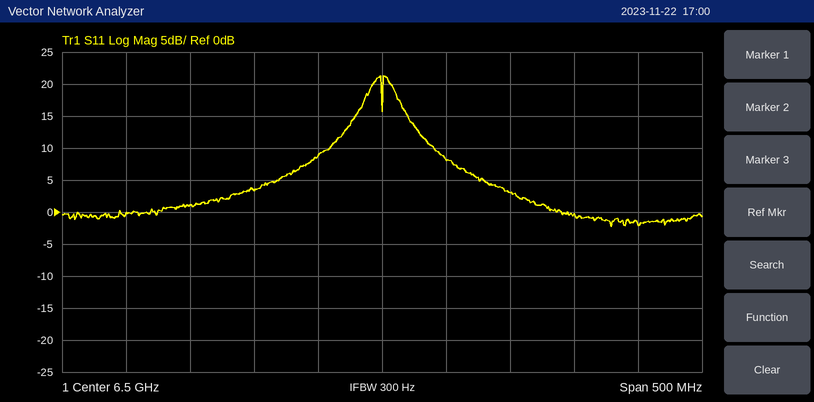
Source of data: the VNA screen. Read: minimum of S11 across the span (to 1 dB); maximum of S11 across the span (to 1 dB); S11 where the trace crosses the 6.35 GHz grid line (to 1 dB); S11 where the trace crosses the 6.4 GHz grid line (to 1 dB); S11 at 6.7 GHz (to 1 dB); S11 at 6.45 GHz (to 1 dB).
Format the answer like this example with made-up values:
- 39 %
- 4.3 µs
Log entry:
- -2 dB
- 21 dB
- 1 dB
- 3 dB
- -2 dB
- 9 dB
